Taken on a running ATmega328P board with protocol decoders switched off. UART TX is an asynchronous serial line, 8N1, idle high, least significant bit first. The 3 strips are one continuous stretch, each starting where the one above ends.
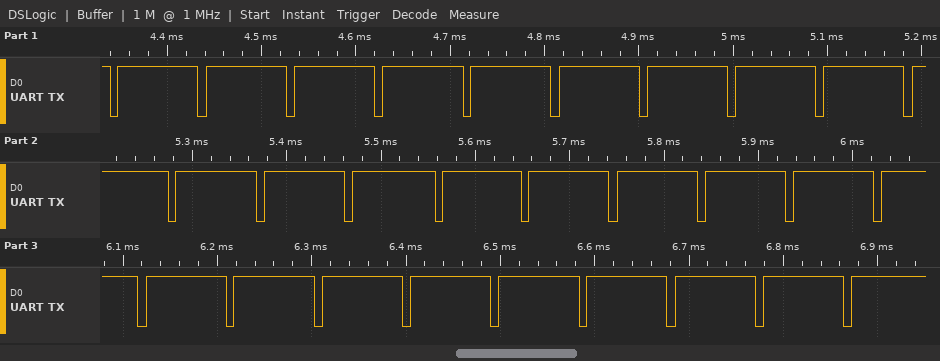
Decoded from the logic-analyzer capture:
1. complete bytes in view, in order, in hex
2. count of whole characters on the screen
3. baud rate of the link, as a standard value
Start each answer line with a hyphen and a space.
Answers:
- FF FF FF FF FF FF FF FF FF FF FF FF FF FF FF FF FF FF FF FF FF FF FF FF FF FF FF FF
- 28
- 115200 baud
